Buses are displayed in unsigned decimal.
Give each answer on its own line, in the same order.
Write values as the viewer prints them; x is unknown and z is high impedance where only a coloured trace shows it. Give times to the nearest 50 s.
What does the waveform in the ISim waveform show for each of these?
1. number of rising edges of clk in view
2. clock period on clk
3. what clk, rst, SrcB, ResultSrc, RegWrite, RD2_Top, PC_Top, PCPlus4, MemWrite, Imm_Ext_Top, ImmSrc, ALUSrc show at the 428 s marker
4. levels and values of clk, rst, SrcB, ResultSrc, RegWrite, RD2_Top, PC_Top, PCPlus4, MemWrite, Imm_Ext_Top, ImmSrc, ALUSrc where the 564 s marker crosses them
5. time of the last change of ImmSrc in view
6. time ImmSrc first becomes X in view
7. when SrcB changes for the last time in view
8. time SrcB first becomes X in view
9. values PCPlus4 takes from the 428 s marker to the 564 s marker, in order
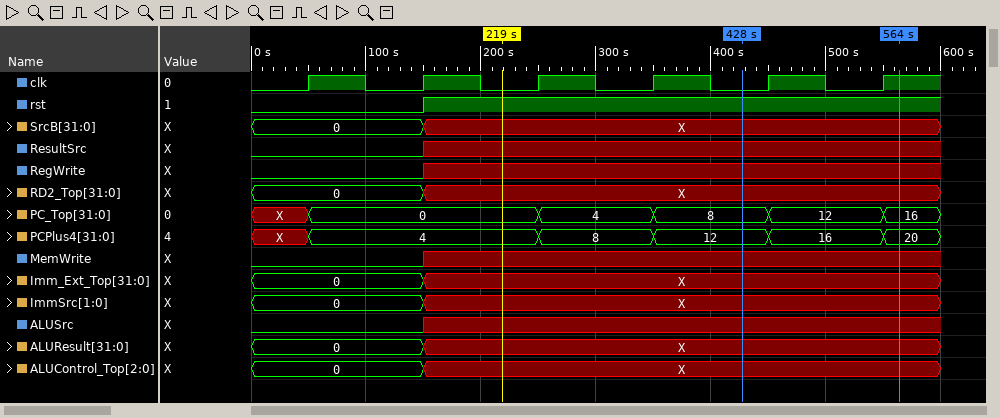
6
100 s
clk=0, rst=1, SrcB=X, ResultSrc=x, RegWrite=x, RD2_Top=X, PC_Top=8, PCPlus4=12, MemWrite=x, Imm_Ext_Top=X, ImmSrc=X, ALUSrc=x
clk=1, rst=1, SrcB=X, ResultSrc=x, RegWrite=x, RD2_Top=X, PC_Top=16, PCPlus4=20, MemWrite=x, Imm_Ext_Top=X, ImmSrc=X, ALUSrc=x
150 s
150 s
150 s
150 s
12, 16, 20
